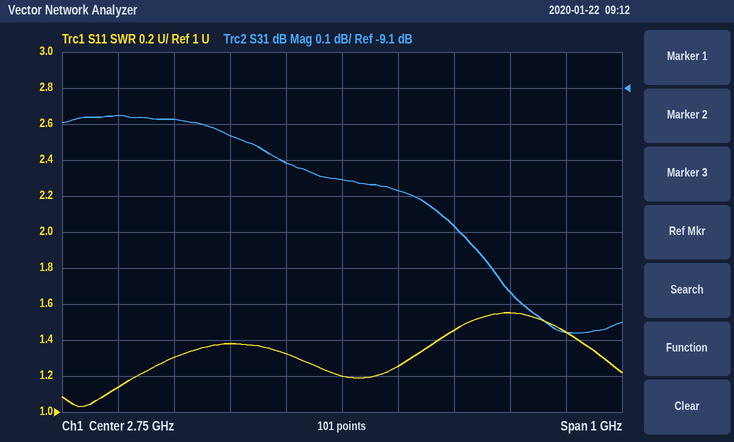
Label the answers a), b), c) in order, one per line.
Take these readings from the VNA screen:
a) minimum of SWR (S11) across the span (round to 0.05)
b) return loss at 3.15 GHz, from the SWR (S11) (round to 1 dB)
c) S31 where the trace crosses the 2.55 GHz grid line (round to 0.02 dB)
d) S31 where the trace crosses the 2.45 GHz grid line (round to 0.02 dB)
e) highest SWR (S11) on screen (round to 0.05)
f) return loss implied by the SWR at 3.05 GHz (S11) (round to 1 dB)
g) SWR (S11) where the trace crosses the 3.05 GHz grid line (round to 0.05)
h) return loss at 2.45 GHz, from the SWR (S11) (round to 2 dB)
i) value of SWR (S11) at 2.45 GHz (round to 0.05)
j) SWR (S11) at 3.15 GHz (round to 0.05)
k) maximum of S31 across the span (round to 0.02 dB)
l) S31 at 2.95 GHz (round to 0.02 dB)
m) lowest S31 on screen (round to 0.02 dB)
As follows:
a) 1.05
b) 15 dB
c) -9.24 dB
d) -9.18 dB
e) 1.55
f) 13 dB
g) 1.55
h) 18 dB
i) 1.30
j) 1.45
k) -9.18 dB
l) -9.48 dB
m) -9.78 dB
